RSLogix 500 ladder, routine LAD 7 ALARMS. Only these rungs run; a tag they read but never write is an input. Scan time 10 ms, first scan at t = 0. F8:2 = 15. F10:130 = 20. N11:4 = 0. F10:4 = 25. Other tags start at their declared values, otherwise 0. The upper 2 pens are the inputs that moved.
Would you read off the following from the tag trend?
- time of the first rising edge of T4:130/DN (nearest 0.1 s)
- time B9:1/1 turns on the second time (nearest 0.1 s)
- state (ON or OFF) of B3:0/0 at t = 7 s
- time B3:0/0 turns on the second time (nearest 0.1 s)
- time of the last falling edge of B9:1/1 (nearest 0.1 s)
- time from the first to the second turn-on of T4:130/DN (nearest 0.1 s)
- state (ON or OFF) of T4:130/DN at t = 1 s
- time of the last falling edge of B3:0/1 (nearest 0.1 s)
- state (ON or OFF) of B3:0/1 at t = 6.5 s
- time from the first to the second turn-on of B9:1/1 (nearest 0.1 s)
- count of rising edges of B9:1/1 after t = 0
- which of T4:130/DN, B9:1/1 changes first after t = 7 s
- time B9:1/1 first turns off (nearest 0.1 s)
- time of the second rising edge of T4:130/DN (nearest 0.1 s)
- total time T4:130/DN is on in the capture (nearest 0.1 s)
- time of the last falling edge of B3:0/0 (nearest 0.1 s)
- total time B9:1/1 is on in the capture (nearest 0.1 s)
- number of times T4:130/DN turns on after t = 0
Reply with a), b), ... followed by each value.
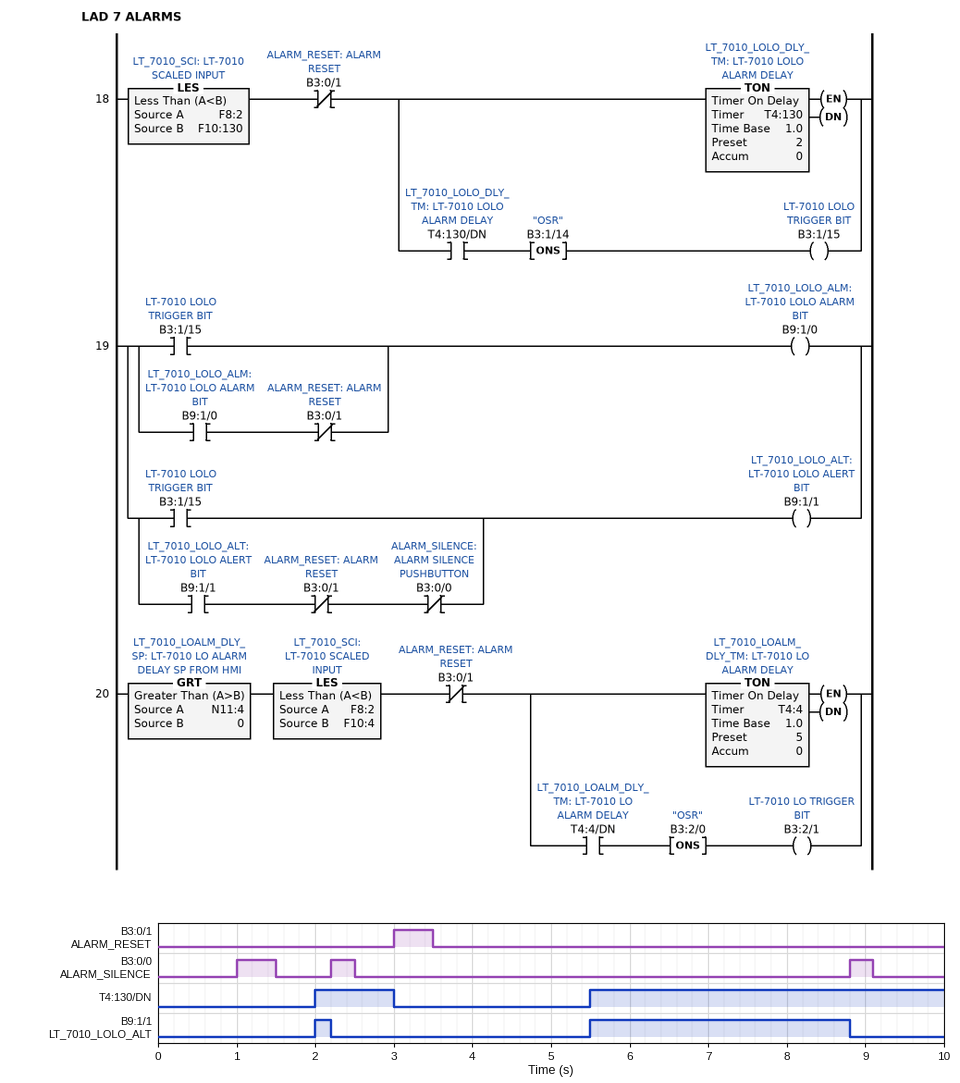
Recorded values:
a) 2.0 s
b) 5.5 s
c) OFF
d) 2.2 s
e) 8.8 s
f) 3.5 s
g) OFF
h) 3.5 s
i) OFF
j) 3.5 s
k) 2
l) B9:1/1
m) 2.2 s
n) 5.5 s
o) 5.5 s
p) 9.1 s
q) 3.5 s
r) 2
